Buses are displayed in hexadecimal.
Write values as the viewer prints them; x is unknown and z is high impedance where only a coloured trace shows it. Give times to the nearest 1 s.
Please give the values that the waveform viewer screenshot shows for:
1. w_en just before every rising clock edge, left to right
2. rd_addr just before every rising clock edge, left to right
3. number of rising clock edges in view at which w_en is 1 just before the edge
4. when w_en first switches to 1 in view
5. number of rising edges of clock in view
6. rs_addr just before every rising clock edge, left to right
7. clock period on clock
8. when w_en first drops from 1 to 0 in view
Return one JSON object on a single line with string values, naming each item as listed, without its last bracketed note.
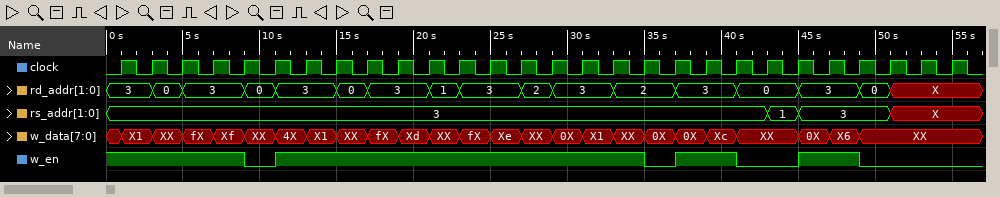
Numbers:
{"w_en just before every rising clock edge, left to right": "1 1 1 1 1 0 1 1 1 1 1 1 1 1 1 1 1 1 0 1 1 0 0 1 1 0 0 0", "rd_addr just before every rising clock edge, left to right": "3, 3, 0, 3, 3, 0, 3, 3, 0, 3, 3, 1, 3, 3, 2, 3, 3, 2, 2, 3, 3, 0, 0, 3, 3, 0, X, X", "number of rising clock edges in view at which w_en is 1 just before the edge": "21", "when w_en first switches to 1 in view": "11 s", "number of rising edges of clock in view": "28", "rs_addr just before every rising clock edge, left to right": "3, 3, 3, 3, 3, 3, 3, 3, 3, 3, 3, 3, 3, 3, 3, 3, 3, 3, 3, 3, 3, 3, 1, 3, 3, 3, X, X", "clock period on clock": "2 s", "when w_en first drops from 1 to 0 in view": "9 s"}
